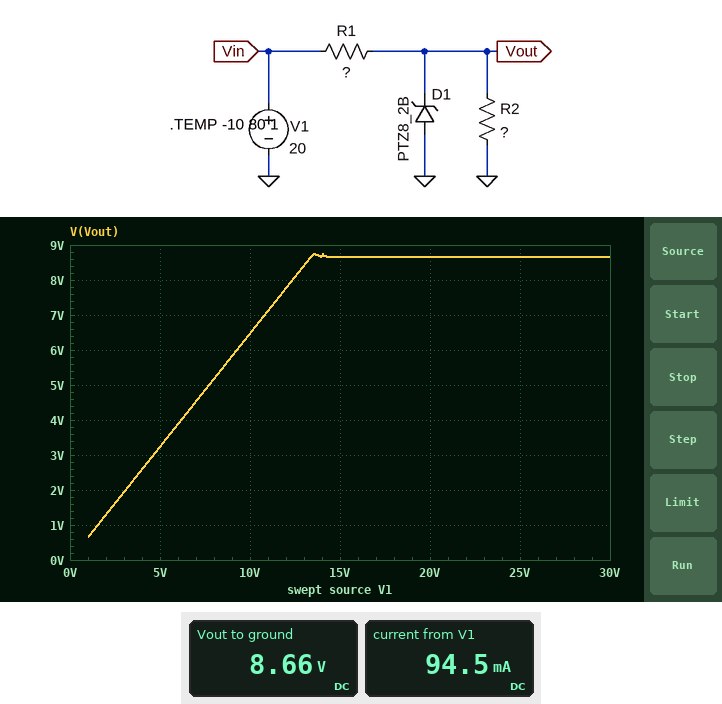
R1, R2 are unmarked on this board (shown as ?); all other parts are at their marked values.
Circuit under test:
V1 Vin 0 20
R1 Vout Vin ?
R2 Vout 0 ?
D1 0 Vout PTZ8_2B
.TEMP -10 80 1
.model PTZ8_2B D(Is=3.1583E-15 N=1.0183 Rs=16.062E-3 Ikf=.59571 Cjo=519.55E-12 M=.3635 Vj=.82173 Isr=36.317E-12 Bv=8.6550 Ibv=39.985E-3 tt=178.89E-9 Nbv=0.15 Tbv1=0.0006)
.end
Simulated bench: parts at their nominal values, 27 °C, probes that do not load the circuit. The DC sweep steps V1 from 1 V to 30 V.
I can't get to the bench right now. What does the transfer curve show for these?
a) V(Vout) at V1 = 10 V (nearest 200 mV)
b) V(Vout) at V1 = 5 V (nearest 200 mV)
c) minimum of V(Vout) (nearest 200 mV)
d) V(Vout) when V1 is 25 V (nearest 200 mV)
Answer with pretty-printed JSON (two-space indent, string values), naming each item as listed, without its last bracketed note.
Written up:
{
  "V(Vout) at V1 = 10 V": "6.4 V",
  "V(Vout) at V1 = 5 V": "3.2 V",
  "minimum of V(Vout)": "600 mV",
  "V(Vout) when V1 is 25 V": "8.6 V"
}
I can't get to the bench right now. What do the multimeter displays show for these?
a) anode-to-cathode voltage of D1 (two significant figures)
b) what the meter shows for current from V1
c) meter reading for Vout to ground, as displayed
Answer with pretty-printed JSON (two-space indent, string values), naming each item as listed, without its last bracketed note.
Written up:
{
  "anode-to-cathode voltage of D1": "-8.7 V",
  "what the meter shows for current from V1": "94.5 mA",
  "meter reading for Vout to ground, as displayed": "8.66 V"
}
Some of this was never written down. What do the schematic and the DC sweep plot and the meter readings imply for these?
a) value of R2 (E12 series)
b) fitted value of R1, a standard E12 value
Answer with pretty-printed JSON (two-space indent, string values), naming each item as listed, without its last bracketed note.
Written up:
{
  "value of R2": "220 Ω",
  "fitted value of R1, a standard E12 value": "120 Ω"
}
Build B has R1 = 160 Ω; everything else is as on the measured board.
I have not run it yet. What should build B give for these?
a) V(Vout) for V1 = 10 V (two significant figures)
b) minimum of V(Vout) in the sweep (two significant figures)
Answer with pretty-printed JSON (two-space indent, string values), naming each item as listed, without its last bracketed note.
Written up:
{
  "V(Vout) for V1 = 10 V": "5.8 V",
  "minimum of V(Vout) in the sweep": "580 mV"
}
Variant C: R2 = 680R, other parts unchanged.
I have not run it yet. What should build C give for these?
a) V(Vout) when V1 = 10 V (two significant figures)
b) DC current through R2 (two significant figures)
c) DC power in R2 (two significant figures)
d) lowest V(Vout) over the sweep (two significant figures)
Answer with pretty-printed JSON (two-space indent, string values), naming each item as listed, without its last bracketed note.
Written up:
{
  "V(Vout) when V1 = 10 V": "8.5 V",
  "DC current through R2": "13 mA",
  "DC power in R2": "110 mW",
  "lowest V(Vout) over the sweep": "850 mV"
}
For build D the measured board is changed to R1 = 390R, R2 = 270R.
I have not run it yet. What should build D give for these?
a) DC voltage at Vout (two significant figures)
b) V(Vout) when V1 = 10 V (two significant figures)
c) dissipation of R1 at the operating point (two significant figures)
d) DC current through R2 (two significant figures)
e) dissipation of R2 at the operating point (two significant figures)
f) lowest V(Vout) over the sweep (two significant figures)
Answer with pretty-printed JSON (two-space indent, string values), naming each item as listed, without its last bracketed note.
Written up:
{
  "DC voltage at Vout": "8.2 V",
  "V(Vout) when V1 = 10 V": "4.1 V",
  "dissipation of R1 at the operating point": "360 mW",
  "DC current through R2": "30 mA",
  "dissipation of R2 at the operating point": "250 mW",
  "lowest V(Vout) over the sweep": "410 mV"
}
